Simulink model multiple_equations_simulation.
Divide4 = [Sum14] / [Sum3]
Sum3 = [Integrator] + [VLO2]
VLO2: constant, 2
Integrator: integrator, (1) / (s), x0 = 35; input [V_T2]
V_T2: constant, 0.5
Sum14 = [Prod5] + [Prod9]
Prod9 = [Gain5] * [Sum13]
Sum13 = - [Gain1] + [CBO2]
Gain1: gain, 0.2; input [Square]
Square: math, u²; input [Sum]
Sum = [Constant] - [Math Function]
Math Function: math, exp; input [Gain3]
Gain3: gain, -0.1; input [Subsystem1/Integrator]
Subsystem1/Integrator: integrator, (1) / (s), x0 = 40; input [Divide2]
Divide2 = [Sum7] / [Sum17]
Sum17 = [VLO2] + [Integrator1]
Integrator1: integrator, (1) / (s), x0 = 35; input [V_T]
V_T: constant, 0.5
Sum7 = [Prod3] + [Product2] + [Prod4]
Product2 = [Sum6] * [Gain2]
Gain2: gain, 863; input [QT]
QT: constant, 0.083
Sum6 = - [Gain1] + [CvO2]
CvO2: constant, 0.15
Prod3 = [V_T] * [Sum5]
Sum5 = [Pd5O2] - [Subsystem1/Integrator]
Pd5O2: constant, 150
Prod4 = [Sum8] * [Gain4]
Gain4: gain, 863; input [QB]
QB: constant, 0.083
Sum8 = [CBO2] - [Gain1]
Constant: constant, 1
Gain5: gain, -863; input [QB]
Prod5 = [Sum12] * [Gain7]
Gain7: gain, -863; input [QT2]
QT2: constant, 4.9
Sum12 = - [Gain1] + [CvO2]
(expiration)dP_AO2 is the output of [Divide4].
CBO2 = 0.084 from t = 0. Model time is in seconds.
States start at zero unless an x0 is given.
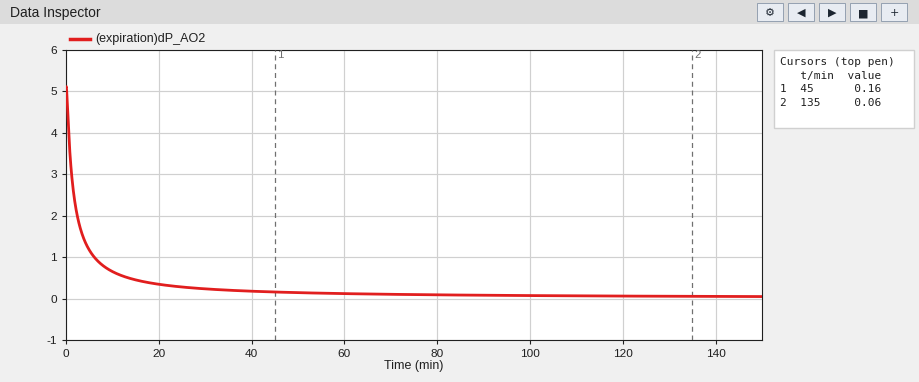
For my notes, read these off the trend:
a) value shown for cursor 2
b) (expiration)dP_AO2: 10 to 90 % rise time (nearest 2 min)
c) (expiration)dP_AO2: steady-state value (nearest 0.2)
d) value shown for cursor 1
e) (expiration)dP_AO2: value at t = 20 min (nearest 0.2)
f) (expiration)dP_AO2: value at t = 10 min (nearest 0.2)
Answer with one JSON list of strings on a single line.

["0.06", "12 min", "0.0", "0.16", "0.4", "0.6"]
